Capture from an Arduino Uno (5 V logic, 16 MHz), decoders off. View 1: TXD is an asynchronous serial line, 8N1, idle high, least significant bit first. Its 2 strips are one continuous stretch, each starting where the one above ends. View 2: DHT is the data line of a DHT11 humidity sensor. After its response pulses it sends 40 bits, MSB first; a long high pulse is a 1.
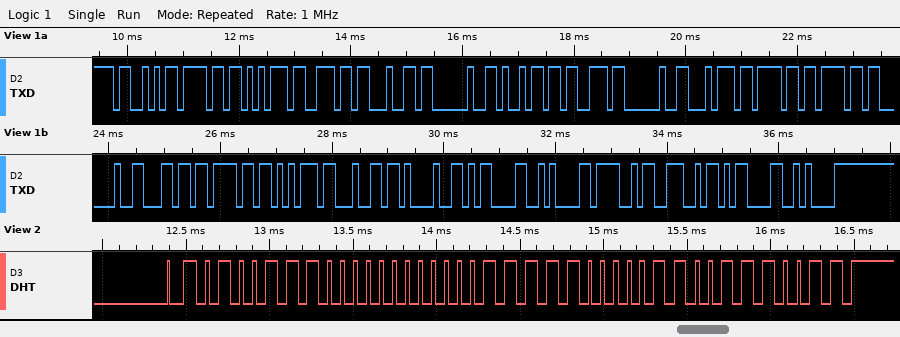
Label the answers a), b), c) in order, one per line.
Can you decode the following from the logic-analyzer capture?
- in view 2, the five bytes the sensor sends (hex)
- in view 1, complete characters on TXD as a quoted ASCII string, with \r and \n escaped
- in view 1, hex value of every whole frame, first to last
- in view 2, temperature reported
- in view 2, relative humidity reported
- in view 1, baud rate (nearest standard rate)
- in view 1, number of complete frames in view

a) 4E 00 1F 06 73
b) "Sound is too loud!\r\nON\r\n"
c) 53 6F 75 6E 64 20 69 73 20 74 6F 6F 20 6C 6F 75 64 21 0D 0A 4F 4E 0D 0A
d) 31.6 °C
e) 78 %
f) 9600 baud
g) 24
